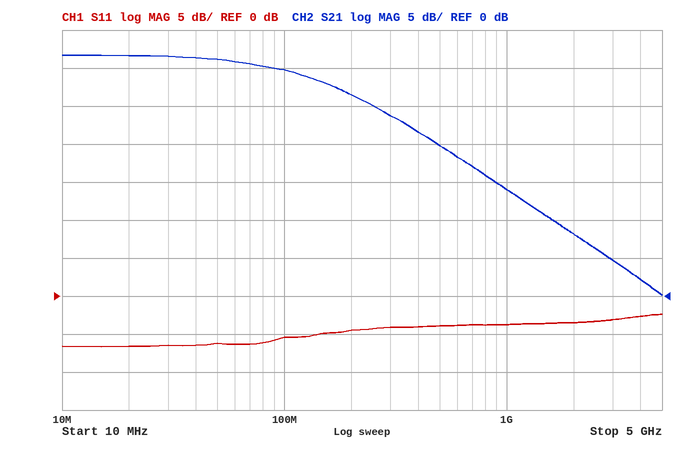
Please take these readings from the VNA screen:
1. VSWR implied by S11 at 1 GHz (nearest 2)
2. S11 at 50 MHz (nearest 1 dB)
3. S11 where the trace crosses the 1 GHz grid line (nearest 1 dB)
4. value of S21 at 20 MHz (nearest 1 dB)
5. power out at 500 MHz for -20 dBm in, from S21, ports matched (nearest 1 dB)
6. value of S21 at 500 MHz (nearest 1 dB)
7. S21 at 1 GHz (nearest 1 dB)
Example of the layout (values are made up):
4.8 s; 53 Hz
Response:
4; -6 dB; -4 dB; 32 dB; 0 dBm; 20 dB; 14 dB
